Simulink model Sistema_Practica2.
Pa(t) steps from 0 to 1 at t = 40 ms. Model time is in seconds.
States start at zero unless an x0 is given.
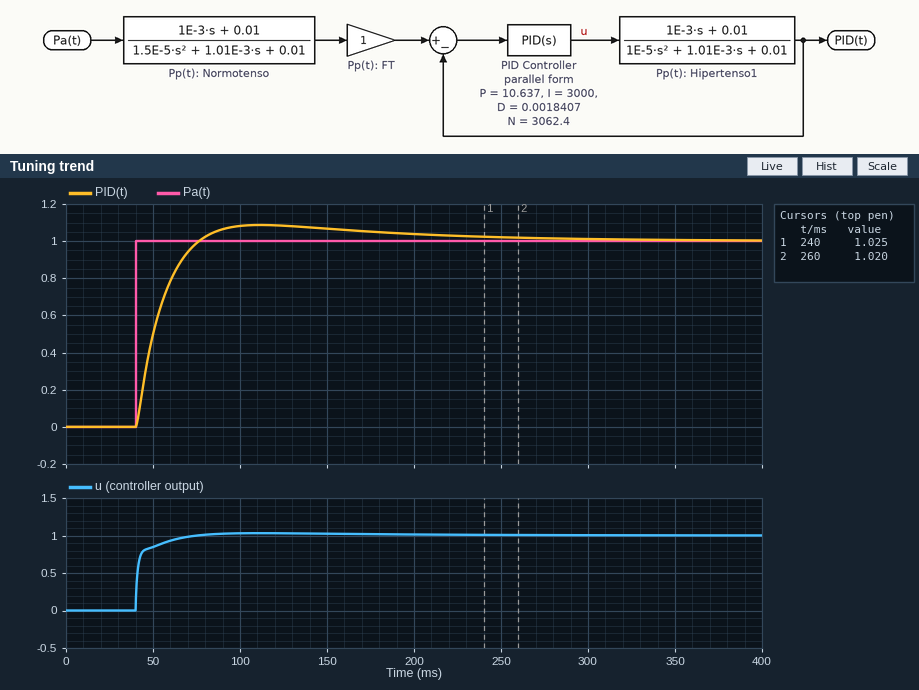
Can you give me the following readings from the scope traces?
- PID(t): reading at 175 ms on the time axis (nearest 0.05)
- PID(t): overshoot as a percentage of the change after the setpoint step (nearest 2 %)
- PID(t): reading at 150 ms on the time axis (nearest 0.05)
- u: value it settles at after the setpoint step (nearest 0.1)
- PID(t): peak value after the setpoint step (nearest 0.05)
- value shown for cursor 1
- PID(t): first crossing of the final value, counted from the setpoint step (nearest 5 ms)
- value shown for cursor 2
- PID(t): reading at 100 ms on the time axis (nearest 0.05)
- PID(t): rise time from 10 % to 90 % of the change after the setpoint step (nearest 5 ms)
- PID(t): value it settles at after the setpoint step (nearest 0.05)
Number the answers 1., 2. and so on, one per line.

1. 1.05
2. 8 %
3. 1.05
4. 1.0
5. 1.10
6. 1.025
7. 35 ms
8. 1.020
9. 1.10
10. 25 ms
11. 1.00
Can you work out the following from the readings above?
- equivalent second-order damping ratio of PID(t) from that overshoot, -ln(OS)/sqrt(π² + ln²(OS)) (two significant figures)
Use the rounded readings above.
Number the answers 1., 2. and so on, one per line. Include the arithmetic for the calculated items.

1. ln(0.08) = -2.526; 2.526 / sqrt(9.870 + 6.379) = 0.63
